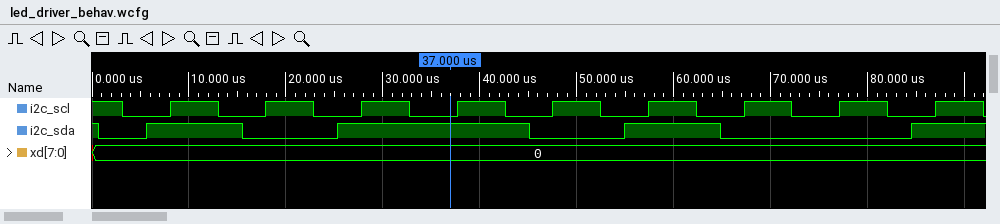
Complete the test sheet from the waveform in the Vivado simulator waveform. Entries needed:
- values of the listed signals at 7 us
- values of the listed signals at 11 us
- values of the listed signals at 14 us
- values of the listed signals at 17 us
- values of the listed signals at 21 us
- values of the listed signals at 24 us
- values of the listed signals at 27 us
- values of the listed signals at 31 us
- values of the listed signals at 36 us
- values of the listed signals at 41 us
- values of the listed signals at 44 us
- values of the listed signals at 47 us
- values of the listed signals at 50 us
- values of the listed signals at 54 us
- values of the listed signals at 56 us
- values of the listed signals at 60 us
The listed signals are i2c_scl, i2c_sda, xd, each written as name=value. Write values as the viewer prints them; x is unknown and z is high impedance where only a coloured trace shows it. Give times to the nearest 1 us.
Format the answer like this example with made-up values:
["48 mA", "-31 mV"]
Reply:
["i2c_scl=0, i2c_sda=1, xd=0", "i2c_scl=1, i2c_sda=1, xd=0", "i2c_scl=0, i2c_sda=1, xd=0", "i2c_scl=0, i2c_sda=0, xd=0", "i2c_scl=1, i2c_sda=0, xd=0", "i2c_scl=0, i2c_sda=0, xd=0", "i2c_scl=0, i2c_sda=1, xd=0", "i2c_scl=1, i2c_sda=1, xd=0", "i2c_scl=0, i2c_sda=1, xd=0", "i2c_scl=1, i2c_sda=1, xd=0", "i2c_scl=0, i2c_sda=1, xd=0", "i2c_scl=0, i2c_sda=0, xd=0", "i2c_scl=1, i2c_sda=0, xd=0", "i2c_scl=0, i2c_sda=0, xd=0", "i2c_scl=0, i2c_sda=1, xd=0", "i2c_scl=1, i2c_sda=1, xd=0"]
